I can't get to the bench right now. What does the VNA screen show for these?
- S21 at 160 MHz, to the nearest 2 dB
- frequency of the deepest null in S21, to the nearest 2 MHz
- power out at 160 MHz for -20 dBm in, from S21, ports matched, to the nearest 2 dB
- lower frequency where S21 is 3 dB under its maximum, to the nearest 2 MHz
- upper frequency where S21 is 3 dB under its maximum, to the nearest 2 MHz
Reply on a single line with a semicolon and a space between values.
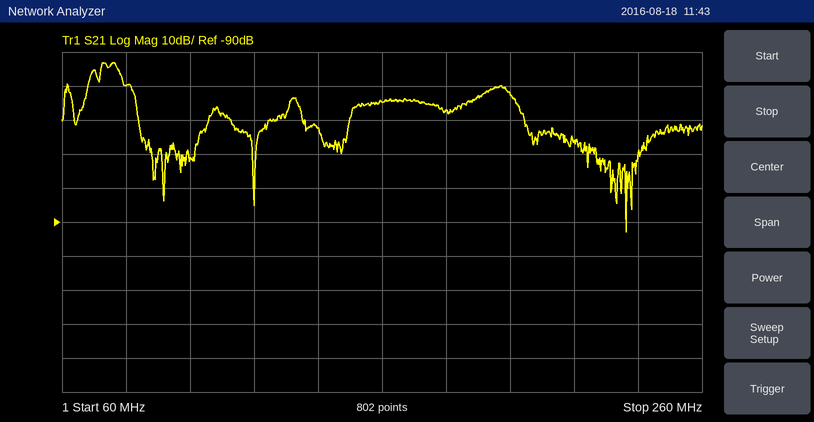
-54 dB; 236 MHz; -74 dBm; 72 MHz; 78 MHz
